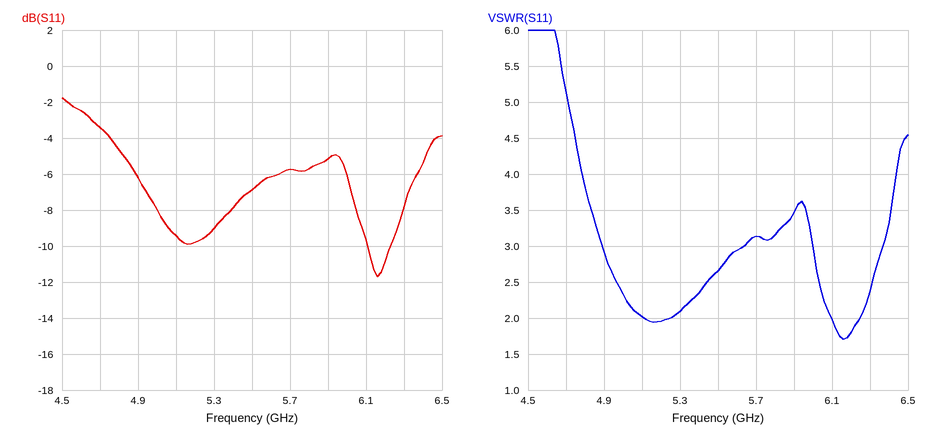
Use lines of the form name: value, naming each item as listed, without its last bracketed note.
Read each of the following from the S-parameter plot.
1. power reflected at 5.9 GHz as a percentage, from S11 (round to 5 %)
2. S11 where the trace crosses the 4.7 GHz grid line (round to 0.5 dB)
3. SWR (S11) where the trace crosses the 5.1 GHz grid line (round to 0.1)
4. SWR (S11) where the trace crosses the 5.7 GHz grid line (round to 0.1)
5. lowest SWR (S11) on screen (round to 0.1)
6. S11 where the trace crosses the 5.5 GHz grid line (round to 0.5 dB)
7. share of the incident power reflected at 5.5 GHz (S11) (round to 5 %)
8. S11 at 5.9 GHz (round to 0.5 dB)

power reflected at 5.9 GHz as a percentage, from S11: 30 %
S11 where the trace crosses the 4.7 GHz grid line: -3.5 dB
SWR (S11) where the trace crosses the 5.1 GHz grid line: 2.0
SWR (S11) where the trace crosses the 5.7 GHz grid line: 3.1
lowest SWR (S11) on screen: 1.7
S11 where the trace crosses the 5.5 GHz grid line: -7.0 dB
share of the incident power reflected at 5.5 GHz (S11): 20 %
S11 at 5.9 GHz: -5.0 dB
